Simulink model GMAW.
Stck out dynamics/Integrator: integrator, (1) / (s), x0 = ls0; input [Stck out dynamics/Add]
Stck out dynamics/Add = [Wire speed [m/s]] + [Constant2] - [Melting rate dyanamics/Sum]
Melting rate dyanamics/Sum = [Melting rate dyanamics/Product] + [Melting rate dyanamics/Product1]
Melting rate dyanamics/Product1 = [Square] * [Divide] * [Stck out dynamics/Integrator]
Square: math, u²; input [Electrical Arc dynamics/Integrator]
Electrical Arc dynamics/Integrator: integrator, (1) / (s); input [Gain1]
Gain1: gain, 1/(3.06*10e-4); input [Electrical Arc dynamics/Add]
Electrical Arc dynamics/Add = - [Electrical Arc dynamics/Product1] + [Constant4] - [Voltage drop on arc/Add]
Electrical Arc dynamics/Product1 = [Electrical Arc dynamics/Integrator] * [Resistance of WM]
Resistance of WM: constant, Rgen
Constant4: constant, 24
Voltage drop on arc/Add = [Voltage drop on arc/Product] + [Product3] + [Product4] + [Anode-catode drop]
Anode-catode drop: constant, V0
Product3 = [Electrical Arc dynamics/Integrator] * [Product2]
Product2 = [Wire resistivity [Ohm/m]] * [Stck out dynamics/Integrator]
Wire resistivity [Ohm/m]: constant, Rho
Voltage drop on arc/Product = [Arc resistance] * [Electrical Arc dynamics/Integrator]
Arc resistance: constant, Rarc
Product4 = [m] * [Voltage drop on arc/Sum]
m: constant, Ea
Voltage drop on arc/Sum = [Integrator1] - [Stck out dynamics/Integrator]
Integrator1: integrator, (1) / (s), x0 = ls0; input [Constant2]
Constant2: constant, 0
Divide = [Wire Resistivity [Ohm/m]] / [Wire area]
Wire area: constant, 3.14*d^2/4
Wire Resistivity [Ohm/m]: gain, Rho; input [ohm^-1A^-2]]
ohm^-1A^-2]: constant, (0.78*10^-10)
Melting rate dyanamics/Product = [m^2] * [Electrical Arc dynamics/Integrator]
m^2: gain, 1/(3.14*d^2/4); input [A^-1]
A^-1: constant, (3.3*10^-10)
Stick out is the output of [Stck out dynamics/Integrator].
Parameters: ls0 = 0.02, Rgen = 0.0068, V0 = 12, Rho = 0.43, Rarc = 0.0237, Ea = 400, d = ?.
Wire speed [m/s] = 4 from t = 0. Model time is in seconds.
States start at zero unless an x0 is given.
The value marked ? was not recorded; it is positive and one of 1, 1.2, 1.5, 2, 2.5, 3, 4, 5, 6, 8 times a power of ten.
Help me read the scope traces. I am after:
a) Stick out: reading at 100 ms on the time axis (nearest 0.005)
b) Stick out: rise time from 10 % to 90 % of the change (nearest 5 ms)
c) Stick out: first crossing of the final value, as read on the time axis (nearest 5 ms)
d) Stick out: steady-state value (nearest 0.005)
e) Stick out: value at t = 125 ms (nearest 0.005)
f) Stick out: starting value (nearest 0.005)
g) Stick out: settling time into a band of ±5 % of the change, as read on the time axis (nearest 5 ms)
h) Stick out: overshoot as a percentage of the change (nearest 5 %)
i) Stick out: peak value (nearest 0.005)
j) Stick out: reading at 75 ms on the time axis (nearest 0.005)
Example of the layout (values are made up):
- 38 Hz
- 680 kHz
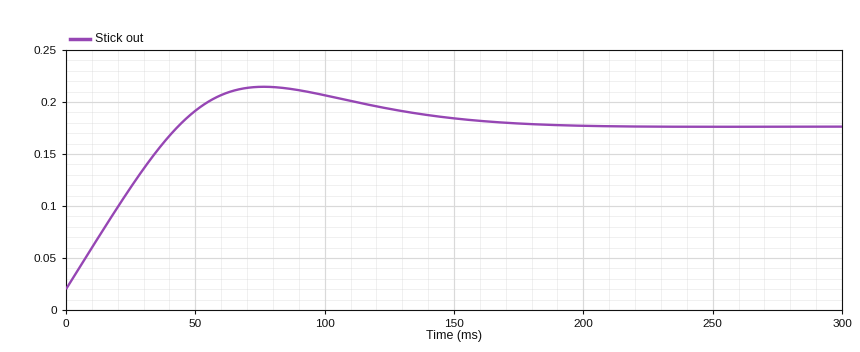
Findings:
- 0.205
- 35 ms
- 45 ms
- 0.175
- 0.195
- 0.020
- 150 ms
- 25 %
- 0.215
- 0.215
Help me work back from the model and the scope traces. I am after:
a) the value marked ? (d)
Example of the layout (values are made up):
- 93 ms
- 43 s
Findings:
- 0.001
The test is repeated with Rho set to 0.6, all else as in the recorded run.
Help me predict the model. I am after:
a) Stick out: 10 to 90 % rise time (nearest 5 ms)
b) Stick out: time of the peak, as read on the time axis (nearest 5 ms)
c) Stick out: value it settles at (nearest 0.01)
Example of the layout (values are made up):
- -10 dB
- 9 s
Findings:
- 45 ms
- 90 ms
- 0.20
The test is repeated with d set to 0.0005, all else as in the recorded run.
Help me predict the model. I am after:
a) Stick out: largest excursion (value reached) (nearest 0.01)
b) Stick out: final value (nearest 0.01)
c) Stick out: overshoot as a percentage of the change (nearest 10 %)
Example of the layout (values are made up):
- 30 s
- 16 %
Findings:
- 0.14
- 0.07
- 150 %
